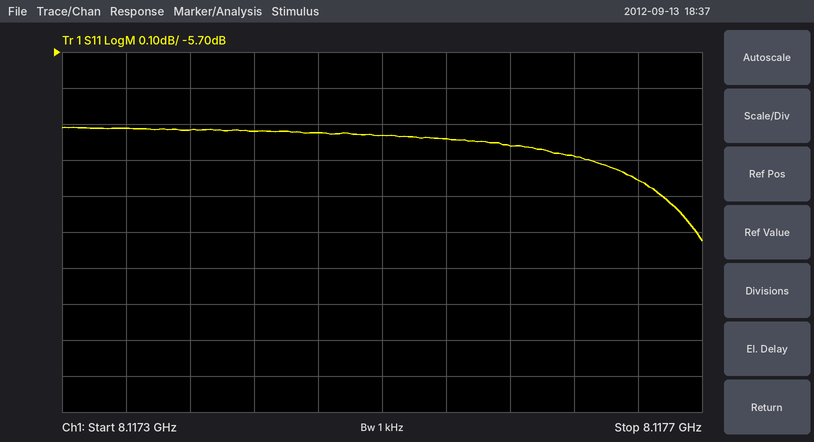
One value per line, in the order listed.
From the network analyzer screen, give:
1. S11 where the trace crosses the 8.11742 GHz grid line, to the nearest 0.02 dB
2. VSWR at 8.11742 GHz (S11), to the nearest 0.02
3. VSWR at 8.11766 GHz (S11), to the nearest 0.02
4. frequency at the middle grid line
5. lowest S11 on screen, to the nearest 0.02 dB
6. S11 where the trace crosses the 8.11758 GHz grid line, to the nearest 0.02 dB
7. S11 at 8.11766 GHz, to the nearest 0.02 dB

-5.92 dB
3.04
2.98
8.1175 GHz
-6.22 dB
-5.96 dB
-6.06 dB
